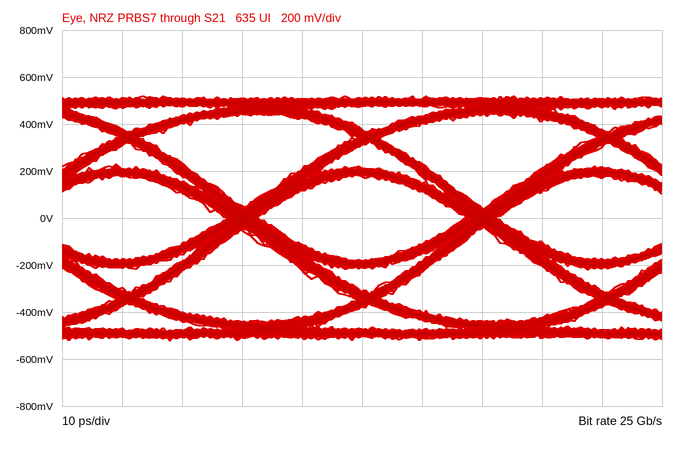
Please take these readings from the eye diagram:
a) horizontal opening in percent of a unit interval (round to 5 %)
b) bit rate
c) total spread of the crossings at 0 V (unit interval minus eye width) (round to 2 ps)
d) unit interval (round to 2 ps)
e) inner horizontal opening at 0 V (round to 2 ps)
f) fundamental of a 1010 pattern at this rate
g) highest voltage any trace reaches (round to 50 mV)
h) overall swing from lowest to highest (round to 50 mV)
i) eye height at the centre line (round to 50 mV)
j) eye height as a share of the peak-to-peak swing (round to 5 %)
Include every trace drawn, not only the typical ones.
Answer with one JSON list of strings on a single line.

["85 %", "25 Gb/s", "6 ps", "40 ps", "34 ps", "12.5 GHz", "500 mV", "1.05 V", "350 mV", "35 %"]
